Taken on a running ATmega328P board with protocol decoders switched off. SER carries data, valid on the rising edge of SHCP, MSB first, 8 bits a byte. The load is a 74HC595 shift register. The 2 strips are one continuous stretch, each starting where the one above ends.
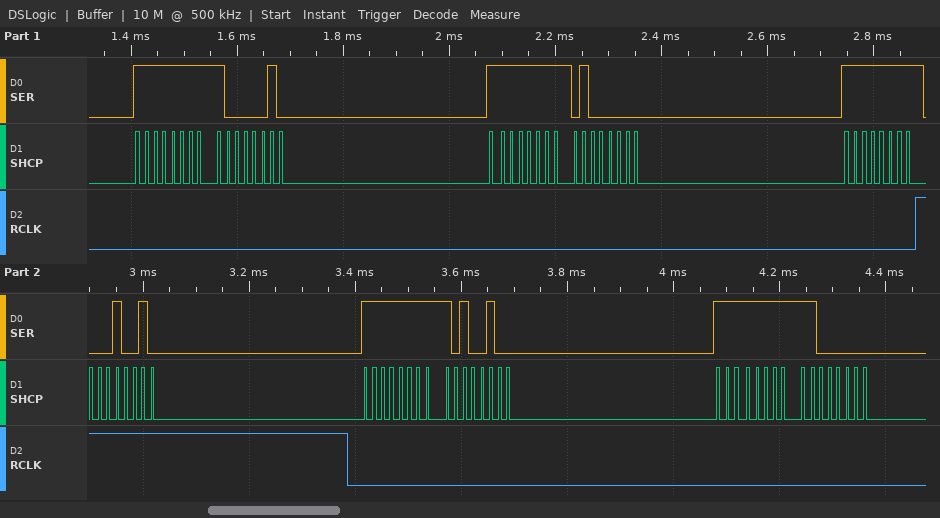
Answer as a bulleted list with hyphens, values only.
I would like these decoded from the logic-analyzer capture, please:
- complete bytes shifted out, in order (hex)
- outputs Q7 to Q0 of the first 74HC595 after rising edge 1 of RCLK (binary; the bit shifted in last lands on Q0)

- FF 82 FF 40 FF 12 FF A4 FF C0
- 11111111
